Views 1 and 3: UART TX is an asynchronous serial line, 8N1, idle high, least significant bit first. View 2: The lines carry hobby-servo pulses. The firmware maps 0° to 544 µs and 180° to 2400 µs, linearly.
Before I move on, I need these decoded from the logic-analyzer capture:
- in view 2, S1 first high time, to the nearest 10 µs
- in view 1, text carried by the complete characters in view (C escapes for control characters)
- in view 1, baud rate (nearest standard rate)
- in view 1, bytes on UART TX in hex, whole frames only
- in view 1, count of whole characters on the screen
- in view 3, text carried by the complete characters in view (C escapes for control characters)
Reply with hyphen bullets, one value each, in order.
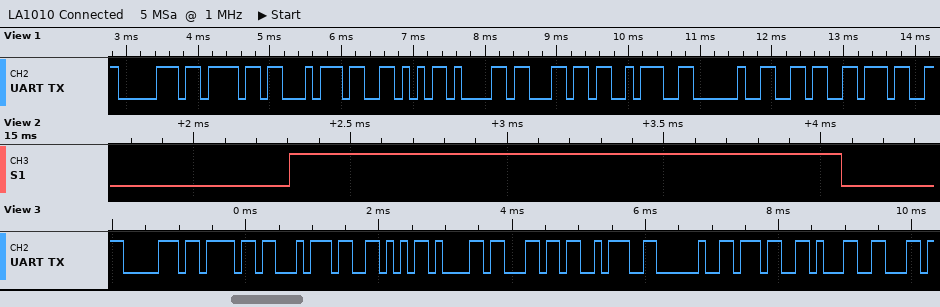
- 1760 µs
- "potVal: 67"
- 9600 baud
- 70 6F 74 56 61 6C 3A 20 36 37
- 10
- "potVal: 71"
